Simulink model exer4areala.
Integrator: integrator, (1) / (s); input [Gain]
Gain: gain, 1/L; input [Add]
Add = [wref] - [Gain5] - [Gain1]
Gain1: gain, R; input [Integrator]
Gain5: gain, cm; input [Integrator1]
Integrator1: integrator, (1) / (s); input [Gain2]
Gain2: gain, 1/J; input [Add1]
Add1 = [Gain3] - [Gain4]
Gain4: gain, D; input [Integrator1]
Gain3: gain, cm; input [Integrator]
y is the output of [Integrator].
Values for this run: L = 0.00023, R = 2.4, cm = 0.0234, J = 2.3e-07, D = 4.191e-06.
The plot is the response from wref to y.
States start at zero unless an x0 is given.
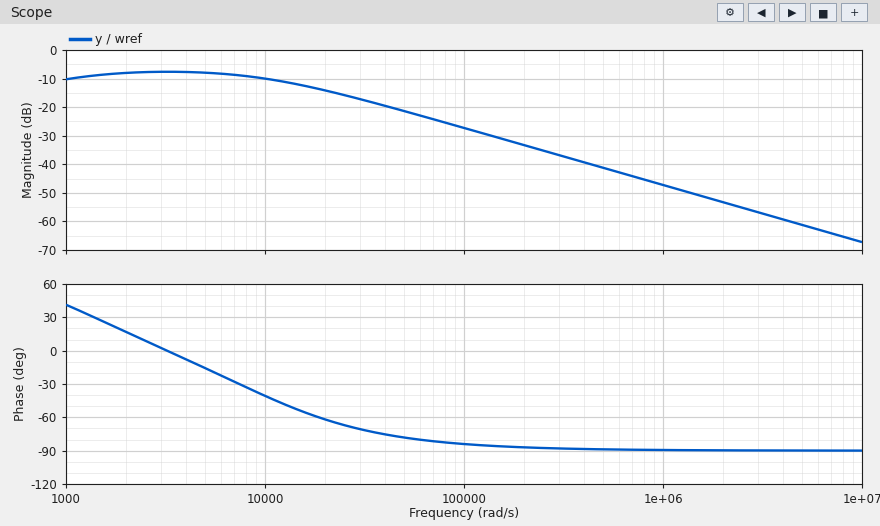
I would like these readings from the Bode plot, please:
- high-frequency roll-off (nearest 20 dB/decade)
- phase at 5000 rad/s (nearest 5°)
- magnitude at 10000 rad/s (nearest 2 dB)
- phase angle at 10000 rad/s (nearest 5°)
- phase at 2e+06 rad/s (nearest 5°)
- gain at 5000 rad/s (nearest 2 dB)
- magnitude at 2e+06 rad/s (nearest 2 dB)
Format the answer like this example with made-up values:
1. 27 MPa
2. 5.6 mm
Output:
1. -20 dB/decade
2. -15°
3. -10 dB
4. -40°
5. -90°
6. -8 dB
7. -54 dB
